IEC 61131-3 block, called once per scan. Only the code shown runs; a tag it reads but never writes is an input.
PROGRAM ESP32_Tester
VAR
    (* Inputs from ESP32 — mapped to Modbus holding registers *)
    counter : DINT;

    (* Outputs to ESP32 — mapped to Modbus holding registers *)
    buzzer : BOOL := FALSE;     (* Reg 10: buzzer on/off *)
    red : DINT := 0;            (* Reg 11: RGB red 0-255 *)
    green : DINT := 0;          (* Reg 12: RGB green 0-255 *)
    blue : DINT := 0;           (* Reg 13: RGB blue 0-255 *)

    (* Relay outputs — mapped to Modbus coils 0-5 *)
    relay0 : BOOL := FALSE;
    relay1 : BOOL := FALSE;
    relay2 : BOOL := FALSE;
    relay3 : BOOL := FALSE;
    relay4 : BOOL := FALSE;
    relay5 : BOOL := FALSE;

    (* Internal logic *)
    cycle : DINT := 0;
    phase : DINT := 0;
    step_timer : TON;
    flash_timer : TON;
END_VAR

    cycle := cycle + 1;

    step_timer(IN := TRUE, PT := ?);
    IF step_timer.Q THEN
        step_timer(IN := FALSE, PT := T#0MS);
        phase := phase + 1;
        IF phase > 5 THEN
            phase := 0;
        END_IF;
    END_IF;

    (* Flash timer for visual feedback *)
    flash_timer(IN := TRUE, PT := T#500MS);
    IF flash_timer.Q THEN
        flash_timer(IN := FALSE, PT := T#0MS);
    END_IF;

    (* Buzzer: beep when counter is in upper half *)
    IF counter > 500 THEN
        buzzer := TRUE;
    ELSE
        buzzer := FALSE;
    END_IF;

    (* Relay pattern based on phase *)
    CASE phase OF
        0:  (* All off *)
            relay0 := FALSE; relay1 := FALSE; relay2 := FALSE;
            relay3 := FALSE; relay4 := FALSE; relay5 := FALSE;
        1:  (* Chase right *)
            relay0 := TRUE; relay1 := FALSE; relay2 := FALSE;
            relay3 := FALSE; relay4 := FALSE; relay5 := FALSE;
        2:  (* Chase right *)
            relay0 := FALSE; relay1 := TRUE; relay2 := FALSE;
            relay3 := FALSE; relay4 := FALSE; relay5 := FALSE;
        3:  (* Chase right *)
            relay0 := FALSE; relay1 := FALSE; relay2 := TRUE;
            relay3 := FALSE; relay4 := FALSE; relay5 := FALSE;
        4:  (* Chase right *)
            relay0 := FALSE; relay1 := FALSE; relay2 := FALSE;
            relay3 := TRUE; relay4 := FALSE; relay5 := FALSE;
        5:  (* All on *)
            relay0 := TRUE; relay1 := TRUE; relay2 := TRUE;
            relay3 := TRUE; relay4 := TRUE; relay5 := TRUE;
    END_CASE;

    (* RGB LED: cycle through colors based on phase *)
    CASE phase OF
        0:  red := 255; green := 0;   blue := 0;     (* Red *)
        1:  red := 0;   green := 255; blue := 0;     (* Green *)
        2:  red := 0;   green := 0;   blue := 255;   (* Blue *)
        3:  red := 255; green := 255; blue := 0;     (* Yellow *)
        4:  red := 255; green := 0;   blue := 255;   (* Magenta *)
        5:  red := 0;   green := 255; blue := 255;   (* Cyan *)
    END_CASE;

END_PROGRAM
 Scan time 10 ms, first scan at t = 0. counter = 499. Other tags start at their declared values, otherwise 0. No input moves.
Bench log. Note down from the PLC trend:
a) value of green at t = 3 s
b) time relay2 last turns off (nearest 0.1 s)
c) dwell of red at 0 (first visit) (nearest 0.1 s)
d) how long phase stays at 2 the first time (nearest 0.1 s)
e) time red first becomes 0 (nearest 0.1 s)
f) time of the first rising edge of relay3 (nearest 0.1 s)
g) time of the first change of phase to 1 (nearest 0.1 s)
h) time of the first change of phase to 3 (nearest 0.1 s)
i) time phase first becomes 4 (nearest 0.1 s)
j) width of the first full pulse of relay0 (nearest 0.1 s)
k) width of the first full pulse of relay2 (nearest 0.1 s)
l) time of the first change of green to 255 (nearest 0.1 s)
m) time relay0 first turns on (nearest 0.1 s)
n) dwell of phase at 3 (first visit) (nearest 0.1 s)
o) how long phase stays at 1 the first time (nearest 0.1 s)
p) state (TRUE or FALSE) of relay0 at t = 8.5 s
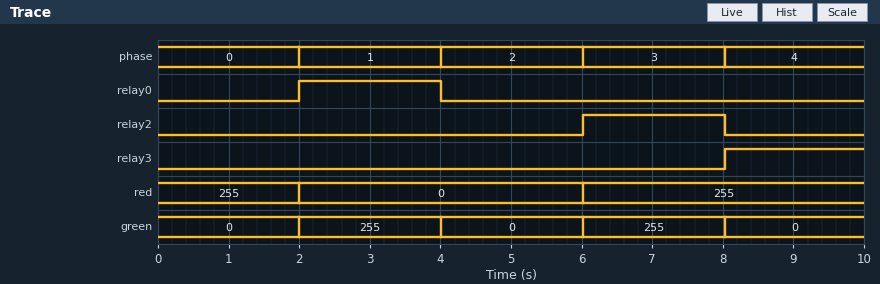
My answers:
255
8.0 s
4.0 s
2.0 s
2.0 s
8.0 s
2.0 s
6.0 s
8.0 s
2.0 s
2.0 s
2.0 s
2.0 s
2.0 s
2.0 s
FALSE
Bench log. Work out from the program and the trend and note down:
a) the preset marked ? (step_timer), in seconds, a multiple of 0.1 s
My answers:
2.0 s
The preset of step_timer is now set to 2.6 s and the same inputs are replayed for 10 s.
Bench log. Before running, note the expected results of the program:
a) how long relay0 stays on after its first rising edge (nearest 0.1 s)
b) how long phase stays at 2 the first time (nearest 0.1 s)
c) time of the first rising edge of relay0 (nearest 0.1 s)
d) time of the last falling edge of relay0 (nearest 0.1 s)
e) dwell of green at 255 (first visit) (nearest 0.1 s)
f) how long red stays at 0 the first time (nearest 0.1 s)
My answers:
2.6 s
2.6 s
2.6 s
5.2 s
2.6 s
5.2 s
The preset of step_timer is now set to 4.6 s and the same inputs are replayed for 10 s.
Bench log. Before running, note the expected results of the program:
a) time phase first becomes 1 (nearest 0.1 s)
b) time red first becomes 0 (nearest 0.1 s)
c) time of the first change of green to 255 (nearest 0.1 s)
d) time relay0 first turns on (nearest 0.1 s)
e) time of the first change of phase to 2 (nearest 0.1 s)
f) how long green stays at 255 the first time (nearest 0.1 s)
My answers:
4.6 s
4.6 s
4.6 s
4.6 s
9.2 s
4.6 s
